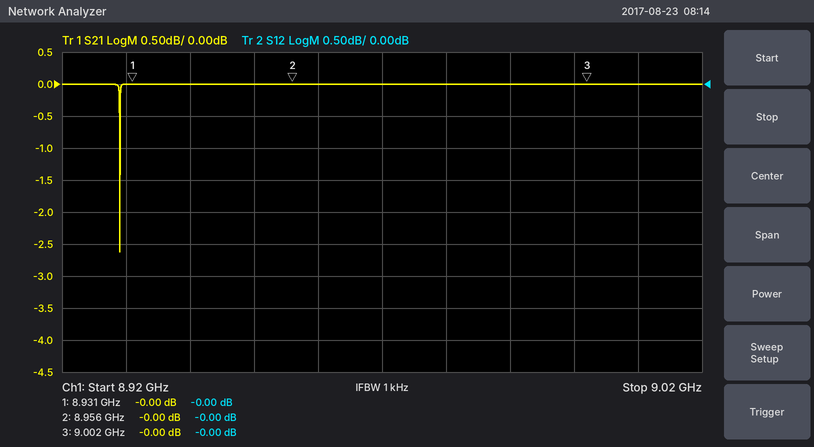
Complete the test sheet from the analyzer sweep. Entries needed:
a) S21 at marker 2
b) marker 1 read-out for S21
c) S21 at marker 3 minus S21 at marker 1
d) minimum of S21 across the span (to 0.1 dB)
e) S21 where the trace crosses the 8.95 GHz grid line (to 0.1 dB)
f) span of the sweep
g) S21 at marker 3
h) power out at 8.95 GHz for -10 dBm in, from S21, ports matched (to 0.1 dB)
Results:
-0.00 dB
-0.00 dB
0.00 dB
-2.6 dB
0.0 dB
100 MHz
-0.00 dB
-10.0 dBm
